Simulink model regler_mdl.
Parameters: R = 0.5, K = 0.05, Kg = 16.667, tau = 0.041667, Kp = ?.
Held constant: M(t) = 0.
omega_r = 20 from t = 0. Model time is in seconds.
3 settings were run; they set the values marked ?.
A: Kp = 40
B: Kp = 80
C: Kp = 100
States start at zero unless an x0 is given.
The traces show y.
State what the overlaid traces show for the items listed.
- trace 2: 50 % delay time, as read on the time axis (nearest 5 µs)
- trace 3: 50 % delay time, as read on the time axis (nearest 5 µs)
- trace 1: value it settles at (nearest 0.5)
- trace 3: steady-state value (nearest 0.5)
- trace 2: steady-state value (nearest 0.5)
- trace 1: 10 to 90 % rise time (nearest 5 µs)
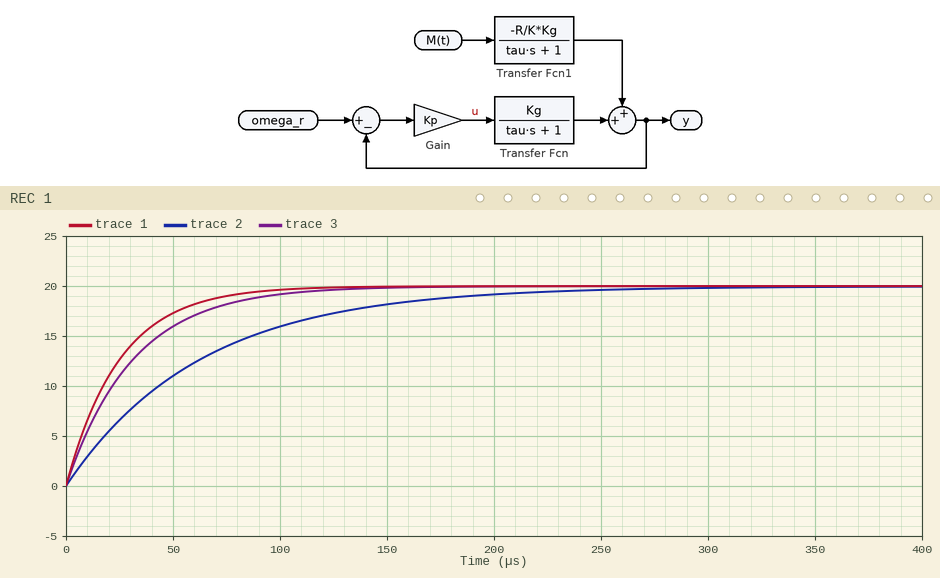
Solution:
45 µs
20 µs
20.0
20.0
20.0
55 µs
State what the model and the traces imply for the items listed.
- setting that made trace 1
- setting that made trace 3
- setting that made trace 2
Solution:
C
B
A
